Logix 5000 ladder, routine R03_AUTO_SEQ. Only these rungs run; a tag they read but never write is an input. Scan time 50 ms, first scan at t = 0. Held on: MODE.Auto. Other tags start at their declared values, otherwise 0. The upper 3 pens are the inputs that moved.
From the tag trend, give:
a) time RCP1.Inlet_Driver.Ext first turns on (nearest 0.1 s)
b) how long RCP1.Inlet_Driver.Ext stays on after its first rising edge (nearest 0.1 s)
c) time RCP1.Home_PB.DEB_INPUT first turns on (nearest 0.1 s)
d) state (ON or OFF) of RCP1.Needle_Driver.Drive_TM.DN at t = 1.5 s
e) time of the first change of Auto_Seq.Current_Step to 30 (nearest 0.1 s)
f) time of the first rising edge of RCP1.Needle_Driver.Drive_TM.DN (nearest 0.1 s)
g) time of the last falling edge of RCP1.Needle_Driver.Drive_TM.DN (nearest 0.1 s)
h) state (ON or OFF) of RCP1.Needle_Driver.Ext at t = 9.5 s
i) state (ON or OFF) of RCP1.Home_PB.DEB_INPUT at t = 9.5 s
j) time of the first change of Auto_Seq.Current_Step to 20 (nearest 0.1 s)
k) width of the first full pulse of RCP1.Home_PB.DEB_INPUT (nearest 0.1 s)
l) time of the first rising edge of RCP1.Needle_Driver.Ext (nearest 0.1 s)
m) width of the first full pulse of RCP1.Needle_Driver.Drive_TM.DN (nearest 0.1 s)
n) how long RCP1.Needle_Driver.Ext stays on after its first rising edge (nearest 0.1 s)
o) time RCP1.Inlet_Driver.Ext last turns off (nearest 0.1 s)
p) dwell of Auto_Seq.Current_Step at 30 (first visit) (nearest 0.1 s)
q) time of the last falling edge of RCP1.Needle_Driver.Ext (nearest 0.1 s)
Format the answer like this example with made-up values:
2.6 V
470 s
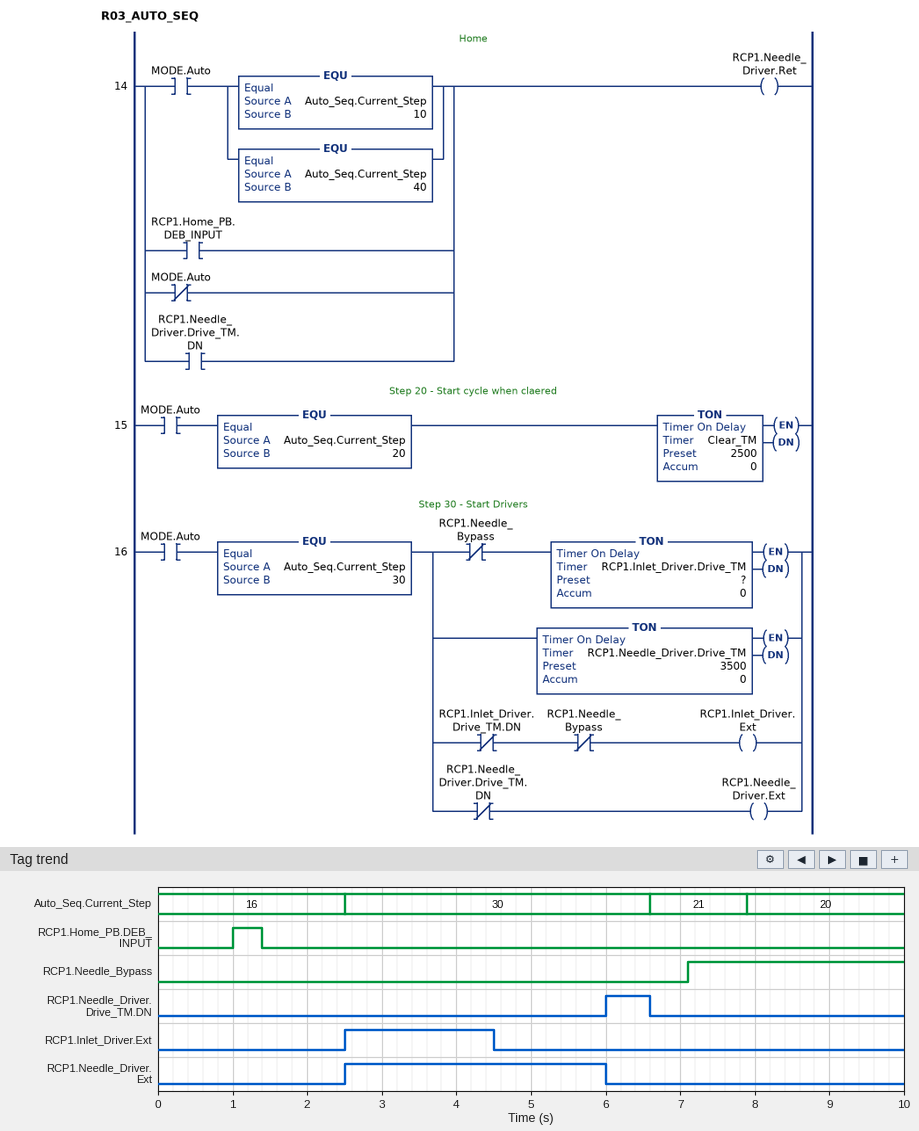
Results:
2.5 s
2.0 s
1.0 s
OFF
2.5 s
6.0 s
6.6 s
OFF
OFF
7.9 s
0.4 s
2.5 s
0.6 s
3.5 s
4.5 s
4.1 s
6.0 s
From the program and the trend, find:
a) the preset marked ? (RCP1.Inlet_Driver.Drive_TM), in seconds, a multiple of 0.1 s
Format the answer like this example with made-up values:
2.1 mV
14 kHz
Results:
2.0 s
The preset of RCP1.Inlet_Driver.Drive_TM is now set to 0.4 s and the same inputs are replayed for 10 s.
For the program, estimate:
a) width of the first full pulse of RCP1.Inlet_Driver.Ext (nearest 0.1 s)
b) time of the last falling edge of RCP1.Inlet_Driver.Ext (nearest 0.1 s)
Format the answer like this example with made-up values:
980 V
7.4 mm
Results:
0.4 s
2.9 s
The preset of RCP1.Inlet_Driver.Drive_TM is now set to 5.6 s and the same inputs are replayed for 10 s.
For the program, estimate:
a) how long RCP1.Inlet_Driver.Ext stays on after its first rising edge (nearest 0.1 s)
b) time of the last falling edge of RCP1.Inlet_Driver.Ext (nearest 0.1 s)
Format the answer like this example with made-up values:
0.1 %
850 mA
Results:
4.1 s
6.6 s
